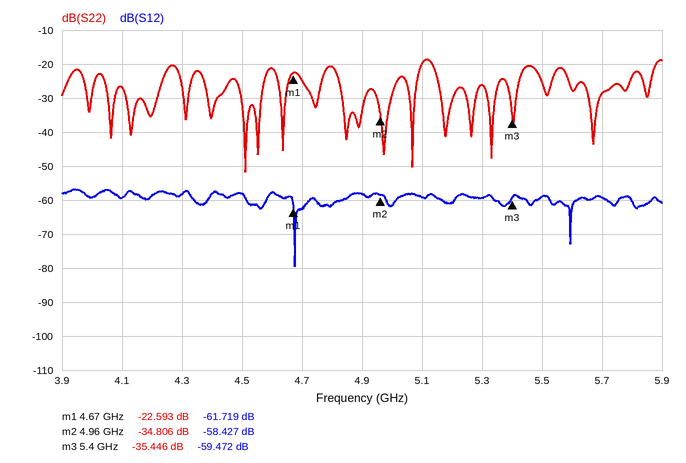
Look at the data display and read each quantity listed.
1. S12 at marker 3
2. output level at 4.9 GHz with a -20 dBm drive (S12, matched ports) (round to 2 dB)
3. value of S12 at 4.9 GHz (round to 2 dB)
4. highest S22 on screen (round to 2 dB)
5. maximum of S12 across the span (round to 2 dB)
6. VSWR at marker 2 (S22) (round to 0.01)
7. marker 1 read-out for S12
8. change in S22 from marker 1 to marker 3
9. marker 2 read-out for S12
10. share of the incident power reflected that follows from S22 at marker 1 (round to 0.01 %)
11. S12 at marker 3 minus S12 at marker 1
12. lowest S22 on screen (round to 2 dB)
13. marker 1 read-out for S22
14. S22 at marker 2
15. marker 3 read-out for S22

-59.472 dB
-78 dBm
-58 dB
-18 dB
-56 dB
1.04
-61.719 dB
-12.853 dB
-58.427 dB
0.55 %
2.247 dB
-52 dB
-22.593 dB
-34.806 dB
-35.446 dB
